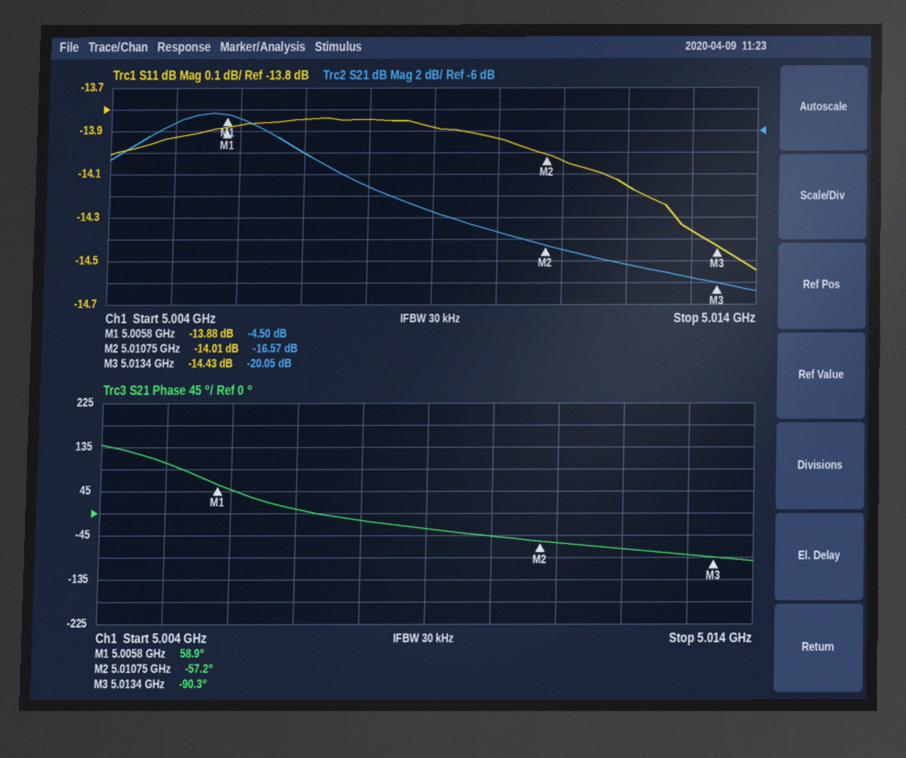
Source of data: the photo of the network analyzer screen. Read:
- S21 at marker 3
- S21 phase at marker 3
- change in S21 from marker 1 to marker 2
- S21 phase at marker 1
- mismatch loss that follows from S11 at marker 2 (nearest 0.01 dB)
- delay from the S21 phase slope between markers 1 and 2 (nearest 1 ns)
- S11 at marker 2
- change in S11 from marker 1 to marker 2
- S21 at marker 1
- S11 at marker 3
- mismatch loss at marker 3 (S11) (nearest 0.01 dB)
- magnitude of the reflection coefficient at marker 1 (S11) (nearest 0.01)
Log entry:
-20.05 dB
-90.3°
-12.07 dB
58.9°
0.18 dB
65 ns
-14.01 dB
-0.13 dB
-4.50 dB
-14.43 dB
0.16 dB
0.20
